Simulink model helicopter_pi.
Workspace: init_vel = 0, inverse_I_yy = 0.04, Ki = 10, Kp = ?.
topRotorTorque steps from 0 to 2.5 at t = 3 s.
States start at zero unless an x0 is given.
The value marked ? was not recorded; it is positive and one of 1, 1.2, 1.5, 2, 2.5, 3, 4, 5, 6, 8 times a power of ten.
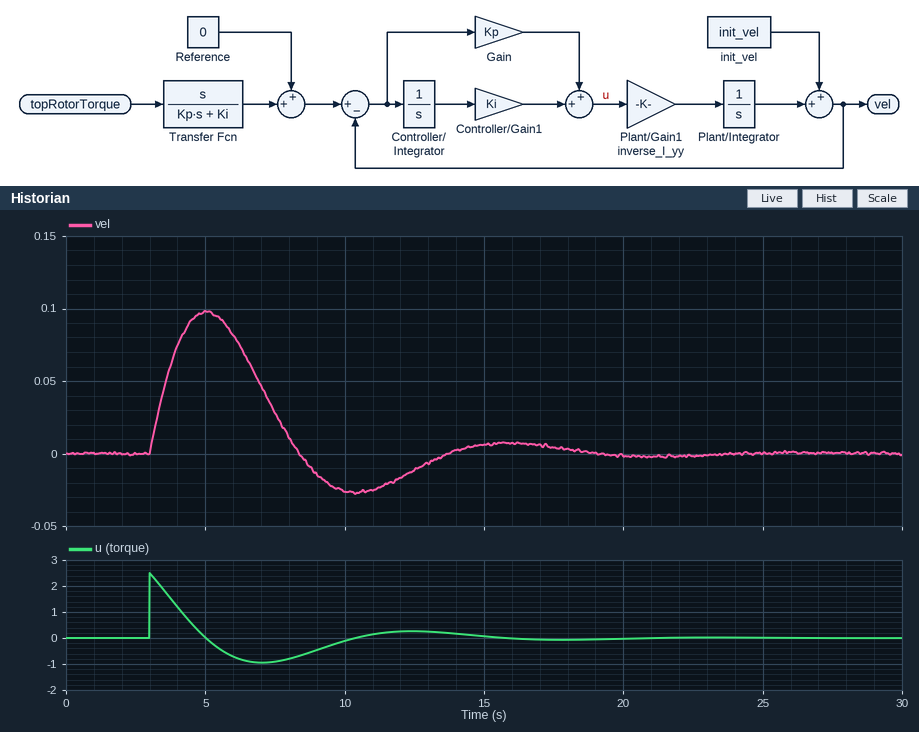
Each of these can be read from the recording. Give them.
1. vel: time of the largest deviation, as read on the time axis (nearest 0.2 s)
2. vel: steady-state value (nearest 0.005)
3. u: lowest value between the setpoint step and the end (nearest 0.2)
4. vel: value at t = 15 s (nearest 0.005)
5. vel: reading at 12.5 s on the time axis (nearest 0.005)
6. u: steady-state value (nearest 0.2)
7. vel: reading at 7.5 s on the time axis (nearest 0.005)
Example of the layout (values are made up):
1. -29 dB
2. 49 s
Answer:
1. 5.0 s
2. 0.000
3. -1.0
4. 0.005
5. -0.010
6. 0.0
7. 0.030
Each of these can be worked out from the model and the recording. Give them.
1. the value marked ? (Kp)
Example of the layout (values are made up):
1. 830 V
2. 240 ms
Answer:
1. 12
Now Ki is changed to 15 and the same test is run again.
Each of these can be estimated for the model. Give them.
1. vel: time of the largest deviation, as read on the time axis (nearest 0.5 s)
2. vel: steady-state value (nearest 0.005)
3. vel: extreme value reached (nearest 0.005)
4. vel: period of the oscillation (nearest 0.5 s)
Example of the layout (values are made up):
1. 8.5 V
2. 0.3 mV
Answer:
1. 4.5 s
2. 0.000
3. 0.085
4. 8.5 s
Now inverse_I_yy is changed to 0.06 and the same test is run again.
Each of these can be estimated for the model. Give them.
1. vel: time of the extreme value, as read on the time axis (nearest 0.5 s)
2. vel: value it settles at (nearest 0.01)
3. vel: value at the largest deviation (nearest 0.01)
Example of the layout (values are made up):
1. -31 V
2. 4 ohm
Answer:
1. 4.5 s
2. 0.00
3. 0.11
